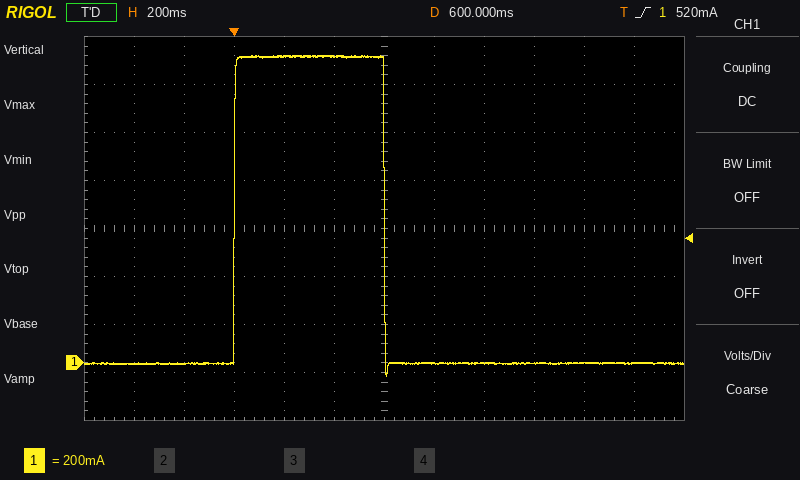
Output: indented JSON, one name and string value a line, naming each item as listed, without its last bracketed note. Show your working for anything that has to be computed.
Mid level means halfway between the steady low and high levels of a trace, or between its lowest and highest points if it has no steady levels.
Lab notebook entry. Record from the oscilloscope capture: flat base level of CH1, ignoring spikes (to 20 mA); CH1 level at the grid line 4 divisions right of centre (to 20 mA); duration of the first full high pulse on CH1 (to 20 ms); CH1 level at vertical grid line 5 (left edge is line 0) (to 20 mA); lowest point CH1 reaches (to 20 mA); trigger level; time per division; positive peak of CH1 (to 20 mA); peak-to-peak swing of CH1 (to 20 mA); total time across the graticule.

{
  "flat base level of CH1, ignoring spikes": "0 mA",
  "CH1 level at the grid line 4 divisions right of centre": "0 mA",
  "duration of the first full high pulse on CH1": "600 ms",
  "CH1 level at vertical grid line 5 (left edge is line 0)": "1.28 A",
  "lowest point CH1 reaches": "-60 mA",
  "trigger level": "520 mA",
  "time per division": "200 ms",
  "positive peak of CH1": "1.28 A",
  "peak-to-peak swing of CH1": "1.28 A − (-60 mA) = 1.34 A",
  "total time across the graticule": "2.4 s"
}
